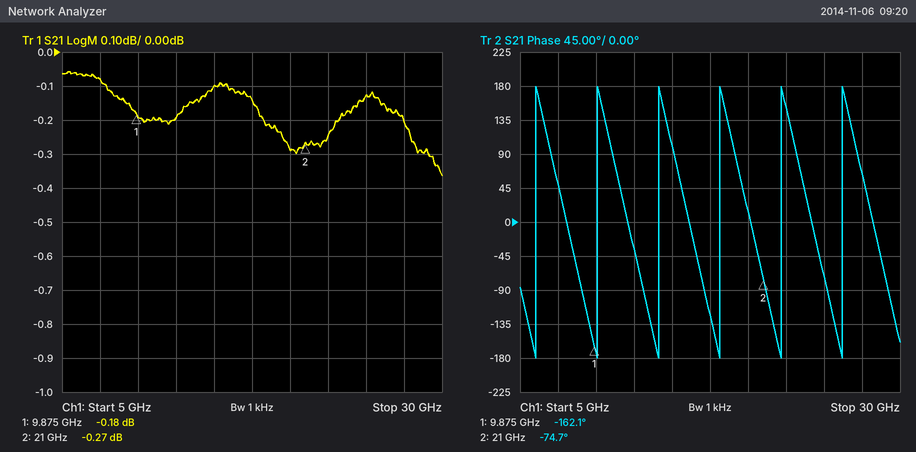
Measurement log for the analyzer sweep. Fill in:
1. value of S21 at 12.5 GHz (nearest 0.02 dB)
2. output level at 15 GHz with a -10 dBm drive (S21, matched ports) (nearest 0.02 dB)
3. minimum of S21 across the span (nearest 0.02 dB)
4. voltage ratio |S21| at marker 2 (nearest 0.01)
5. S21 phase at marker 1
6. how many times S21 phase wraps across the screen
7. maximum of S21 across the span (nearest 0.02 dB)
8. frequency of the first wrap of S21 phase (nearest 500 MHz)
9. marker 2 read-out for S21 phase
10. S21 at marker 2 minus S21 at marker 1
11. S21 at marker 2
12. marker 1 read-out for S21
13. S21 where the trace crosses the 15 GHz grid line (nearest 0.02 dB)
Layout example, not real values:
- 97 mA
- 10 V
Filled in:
- -0.20 dB
- -10.10 dBm
- -0.36 dB
- 0.97
- -162.1°
- 6
- -0.06 dB
- 6.0 GHz
- -74.7°
- -0.09 dB
- -0.27 dB
- -0.18 dB
- -0.10 dB
